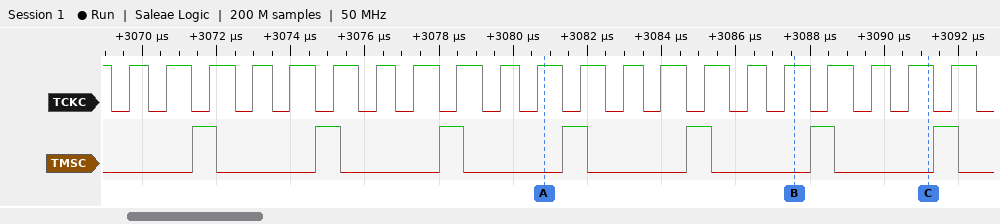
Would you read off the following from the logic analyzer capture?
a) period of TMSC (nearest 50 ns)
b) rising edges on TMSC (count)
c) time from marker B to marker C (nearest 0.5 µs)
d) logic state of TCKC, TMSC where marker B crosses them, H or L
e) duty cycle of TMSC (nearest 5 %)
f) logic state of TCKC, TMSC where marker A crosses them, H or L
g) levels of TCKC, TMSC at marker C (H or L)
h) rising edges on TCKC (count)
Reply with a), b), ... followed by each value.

a) 3350 ns
b) 7
c) 3.5 µs
d) TCKC=H, TMSC=L
e) 20 %
f) TCKC=H, TMSC=L
g) TCKC=H, TMSC=L
h) 21
